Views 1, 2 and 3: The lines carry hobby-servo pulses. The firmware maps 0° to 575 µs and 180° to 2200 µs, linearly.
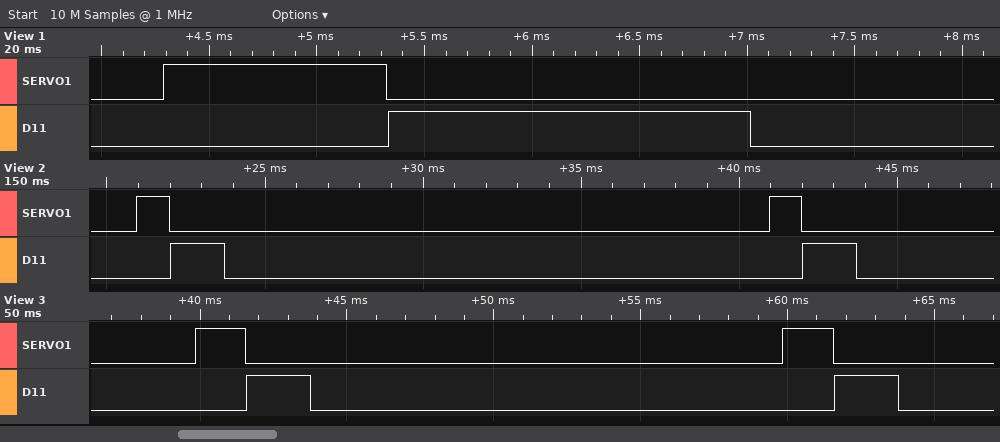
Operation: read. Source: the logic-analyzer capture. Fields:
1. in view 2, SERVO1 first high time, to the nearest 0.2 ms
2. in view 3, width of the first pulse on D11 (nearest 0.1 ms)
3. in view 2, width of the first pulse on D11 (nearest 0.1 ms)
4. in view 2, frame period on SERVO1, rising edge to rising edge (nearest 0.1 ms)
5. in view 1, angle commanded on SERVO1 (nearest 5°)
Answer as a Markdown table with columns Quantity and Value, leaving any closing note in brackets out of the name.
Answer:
| Quantity | Value |
|---|---|
| in view 2, SERVO1 first high time, to the nearest 0.2 ms | 1.0 ms |
| in view 3, width of the first pulse on D11 | 2.2 ms |
| in view 2, width of the first pulse on D11 | 1.7 ms |
| in view 2, frame period on SERVO1, rising edge to rising edge | 20.0 ms |
| in view 1, angle commanded on SERVO1 | 50° |
